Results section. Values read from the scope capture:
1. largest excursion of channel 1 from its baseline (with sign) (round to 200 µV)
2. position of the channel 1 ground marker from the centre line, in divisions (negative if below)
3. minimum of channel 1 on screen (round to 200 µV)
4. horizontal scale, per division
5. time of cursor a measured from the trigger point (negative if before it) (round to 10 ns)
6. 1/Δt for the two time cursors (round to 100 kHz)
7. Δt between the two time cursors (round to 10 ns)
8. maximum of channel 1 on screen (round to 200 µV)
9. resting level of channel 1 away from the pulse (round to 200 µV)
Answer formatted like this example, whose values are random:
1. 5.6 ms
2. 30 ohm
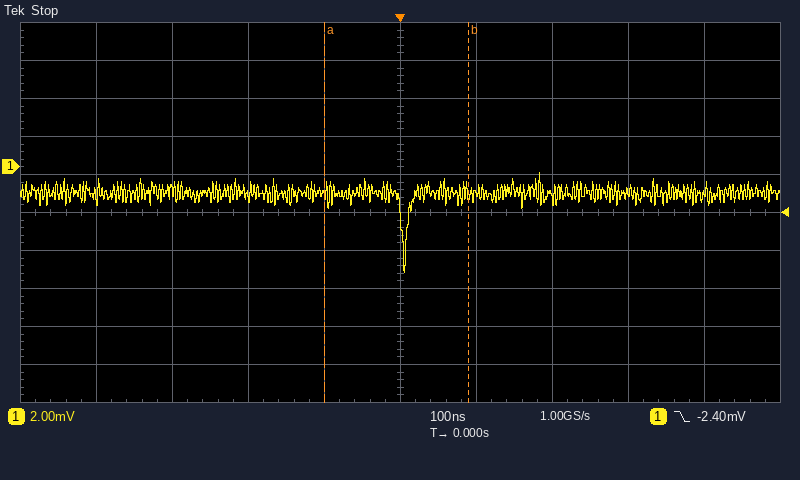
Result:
1. -4.2 mV
2. +1.2 div
3. -5.6 mV
4. 100 ns
5. -100 ns
6. 5.3 MHz
7. 190 ns
8. -200 µV
9. -1.4 mV
